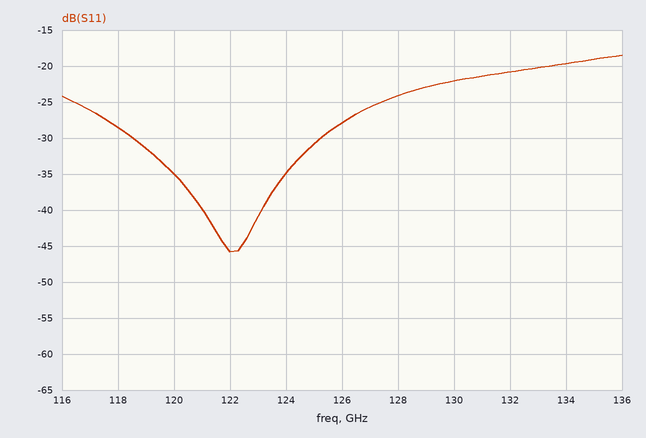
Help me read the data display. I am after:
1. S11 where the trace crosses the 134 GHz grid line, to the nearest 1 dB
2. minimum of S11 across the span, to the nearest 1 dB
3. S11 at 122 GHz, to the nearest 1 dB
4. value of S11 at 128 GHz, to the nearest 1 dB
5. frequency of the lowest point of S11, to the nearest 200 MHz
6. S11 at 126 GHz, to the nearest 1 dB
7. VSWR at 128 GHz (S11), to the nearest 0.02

-20 dB
-46 dB
-46 dB
-24 dB
122.0 GHz
-28 dB
1.14
